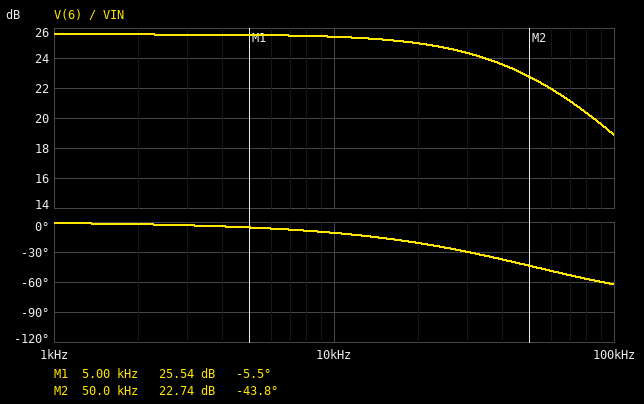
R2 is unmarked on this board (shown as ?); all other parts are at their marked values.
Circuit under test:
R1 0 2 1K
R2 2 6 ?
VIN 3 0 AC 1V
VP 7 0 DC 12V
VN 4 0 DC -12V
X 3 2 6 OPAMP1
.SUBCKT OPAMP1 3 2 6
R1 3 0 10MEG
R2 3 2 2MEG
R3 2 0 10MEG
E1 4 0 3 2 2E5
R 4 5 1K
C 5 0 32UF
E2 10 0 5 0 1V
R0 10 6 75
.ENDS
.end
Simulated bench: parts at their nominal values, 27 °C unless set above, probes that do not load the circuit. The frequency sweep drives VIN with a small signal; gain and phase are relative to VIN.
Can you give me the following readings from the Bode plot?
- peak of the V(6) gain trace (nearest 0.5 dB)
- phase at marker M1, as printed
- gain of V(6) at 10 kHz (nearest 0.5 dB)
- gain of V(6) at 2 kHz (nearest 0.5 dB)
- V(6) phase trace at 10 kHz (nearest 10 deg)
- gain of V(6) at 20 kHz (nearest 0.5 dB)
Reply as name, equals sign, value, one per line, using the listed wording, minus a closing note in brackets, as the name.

peak of the V(6) gain trace = 25.5 dB
phase at marker M1, as printed = -5.5 deg
gain of V(6) at 10 kHz = 25.5 dB
gain of V(6) at 2 kHz = 25.5 dB
V(6) phase trace at 10 kHz = -10 deg
gain of V(6) at 20 kHz = 25.0 dB
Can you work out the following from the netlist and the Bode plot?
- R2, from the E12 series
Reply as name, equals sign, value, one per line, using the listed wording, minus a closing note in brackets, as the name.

R2, from the E12 series = 18 kΩ
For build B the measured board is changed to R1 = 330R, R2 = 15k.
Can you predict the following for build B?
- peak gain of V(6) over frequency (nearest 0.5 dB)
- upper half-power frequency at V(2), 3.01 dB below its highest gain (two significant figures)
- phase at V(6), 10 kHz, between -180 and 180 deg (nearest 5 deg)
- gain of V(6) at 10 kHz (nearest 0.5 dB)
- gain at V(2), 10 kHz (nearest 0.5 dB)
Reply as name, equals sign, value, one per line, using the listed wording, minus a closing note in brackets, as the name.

peak gain of V(6) over frequency = 33.5 dB
upper half-power frequency at V(2), 3.01 dB below its highest gain = 21 kHz
phase at V(6), 10 kHz, between -180 and 180 deg = -25 deg
gain of V(6) at 10 kHz = 32.5 dB
gain at V(2), 10 kHz = -1.0 dB
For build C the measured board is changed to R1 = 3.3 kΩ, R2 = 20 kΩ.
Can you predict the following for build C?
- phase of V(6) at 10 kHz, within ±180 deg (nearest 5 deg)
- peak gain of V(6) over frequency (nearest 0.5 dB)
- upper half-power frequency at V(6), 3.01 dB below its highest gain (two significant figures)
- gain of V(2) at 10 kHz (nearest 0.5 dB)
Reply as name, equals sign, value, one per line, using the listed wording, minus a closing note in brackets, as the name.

phase of V(6) at 10 kHz, within ±180 deg = -5 deg
peak gain of V(6) over frequency = 17.0 dB
upper half-power frequency at V(6), 3.01 dB below its highest gain = 140 kHz
gain of V(2) at 10 kHz = 0 dB
